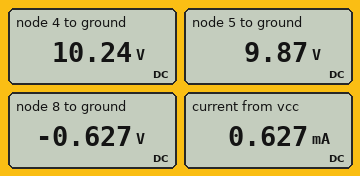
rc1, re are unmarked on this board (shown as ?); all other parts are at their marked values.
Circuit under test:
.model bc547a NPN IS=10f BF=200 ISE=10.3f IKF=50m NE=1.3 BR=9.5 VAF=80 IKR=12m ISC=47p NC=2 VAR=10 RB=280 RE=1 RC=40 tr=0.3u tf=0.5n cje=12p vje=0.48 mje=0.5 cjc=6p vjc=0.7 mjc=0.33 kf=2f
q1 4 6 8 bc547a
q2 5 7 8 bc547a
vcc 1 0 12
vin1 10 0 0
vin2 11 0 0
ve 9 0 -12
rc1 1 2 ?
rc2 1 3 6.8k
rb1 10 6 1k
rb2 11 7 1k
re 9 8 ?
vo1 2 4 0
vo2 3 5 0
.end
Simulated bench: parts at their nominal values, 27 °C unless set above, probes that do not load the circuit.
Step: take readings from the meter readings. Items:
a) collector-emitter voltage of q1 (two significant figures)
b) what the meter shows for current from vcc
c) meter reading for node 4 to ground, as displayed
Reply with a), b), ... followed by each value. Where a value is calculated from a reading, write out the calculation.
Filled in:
a) 10.24 V - (-627 mV) = 11 V
b) 0.627 mA
c) 10.24 V
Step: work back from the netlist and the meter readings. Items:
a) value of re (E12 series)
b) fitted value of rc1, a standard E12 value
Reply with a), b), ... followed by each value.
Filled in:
a) 18 kΩ
b) 5.6 kΩ
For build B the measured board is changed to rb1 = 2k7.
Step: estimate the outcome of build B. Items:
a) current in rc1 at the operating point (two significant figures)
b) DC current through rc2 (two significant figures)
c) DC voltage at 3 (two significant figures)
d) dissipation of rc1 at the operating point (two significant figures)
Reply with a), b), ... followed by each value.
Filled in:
a) 290 µA
b) 330 µA
c) 9.7 V
d) 480 µW
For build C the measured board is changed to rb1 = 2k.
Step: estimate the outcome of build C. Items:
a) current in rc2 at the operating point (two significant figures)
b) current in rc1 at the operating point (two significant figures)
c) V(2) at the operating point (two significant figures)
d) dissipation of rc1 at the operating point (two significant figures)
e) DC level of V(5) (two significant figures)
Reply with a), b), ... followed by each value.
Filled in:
a) 330 µA
b) 300 µA
c) 10 V
d) 510 µW
e) 9.8 V
